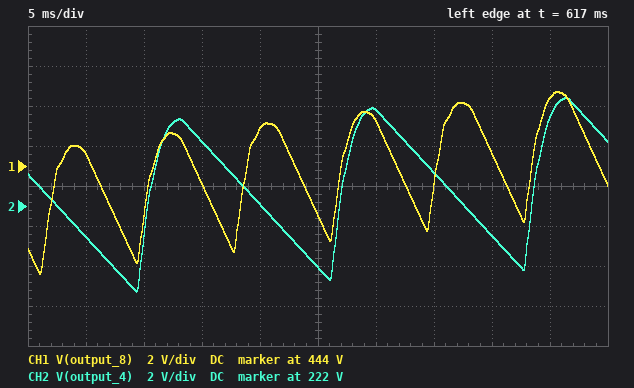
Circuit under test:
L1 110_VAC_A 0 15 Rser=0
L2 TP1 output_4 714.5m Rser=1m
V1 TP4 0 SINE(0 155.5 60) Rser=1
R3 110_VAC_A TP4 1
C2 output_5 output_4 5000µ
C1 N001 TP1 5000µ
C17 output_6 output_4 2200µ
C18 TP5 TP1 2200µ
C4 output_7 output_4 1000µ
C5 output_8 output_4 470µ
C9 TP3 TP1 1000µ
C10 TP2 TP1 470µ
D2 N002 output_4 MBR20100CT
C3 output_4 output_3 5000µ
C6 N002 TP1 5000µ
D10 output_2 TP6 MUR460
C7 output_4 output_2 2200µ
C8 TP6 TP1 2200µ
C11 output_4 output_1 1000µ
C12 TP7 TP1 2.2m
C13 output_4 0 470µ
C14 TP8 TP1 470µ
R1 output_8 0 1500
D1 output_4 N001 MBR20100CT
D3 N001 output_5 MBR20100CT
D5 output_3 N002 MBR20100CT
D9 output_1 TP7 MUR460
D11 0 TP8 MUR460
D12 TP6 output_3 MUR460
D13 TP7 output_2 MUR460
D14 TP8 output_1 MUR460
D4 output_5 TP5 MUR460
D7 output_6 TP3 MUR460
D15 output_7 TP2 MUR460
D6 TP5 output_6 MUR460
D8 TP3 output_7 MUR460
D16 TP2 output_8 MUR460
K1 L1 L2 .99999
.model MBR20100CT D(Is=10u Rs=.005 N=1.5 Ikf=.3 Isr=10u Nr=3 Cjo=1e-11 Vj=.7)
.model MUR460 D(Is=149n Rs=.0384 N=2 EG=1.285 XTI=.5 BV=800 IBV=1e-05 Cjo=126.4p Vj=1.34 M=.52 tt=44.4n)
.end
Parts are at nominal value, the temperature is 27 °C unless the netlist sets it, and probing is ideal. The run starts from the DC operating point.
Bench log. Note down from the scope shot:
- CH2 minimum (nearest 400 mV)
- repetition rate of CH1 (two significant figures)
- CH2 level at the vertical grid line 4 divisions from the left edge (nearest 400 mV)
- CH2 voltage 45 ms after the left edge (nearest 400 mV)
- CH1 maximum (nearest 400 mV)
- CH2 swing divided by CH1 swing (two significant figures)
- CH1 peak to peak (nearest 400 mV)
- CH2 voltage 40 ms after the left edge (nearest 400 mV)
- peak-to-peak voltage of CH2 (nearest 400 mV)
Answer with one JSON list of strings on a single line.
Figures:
["217.6 V", "120 Hz", "222.0 V", "226.4 V", "447.6 V", "1.1", "9.2 V", "220.4 V", "9.6 V"]
